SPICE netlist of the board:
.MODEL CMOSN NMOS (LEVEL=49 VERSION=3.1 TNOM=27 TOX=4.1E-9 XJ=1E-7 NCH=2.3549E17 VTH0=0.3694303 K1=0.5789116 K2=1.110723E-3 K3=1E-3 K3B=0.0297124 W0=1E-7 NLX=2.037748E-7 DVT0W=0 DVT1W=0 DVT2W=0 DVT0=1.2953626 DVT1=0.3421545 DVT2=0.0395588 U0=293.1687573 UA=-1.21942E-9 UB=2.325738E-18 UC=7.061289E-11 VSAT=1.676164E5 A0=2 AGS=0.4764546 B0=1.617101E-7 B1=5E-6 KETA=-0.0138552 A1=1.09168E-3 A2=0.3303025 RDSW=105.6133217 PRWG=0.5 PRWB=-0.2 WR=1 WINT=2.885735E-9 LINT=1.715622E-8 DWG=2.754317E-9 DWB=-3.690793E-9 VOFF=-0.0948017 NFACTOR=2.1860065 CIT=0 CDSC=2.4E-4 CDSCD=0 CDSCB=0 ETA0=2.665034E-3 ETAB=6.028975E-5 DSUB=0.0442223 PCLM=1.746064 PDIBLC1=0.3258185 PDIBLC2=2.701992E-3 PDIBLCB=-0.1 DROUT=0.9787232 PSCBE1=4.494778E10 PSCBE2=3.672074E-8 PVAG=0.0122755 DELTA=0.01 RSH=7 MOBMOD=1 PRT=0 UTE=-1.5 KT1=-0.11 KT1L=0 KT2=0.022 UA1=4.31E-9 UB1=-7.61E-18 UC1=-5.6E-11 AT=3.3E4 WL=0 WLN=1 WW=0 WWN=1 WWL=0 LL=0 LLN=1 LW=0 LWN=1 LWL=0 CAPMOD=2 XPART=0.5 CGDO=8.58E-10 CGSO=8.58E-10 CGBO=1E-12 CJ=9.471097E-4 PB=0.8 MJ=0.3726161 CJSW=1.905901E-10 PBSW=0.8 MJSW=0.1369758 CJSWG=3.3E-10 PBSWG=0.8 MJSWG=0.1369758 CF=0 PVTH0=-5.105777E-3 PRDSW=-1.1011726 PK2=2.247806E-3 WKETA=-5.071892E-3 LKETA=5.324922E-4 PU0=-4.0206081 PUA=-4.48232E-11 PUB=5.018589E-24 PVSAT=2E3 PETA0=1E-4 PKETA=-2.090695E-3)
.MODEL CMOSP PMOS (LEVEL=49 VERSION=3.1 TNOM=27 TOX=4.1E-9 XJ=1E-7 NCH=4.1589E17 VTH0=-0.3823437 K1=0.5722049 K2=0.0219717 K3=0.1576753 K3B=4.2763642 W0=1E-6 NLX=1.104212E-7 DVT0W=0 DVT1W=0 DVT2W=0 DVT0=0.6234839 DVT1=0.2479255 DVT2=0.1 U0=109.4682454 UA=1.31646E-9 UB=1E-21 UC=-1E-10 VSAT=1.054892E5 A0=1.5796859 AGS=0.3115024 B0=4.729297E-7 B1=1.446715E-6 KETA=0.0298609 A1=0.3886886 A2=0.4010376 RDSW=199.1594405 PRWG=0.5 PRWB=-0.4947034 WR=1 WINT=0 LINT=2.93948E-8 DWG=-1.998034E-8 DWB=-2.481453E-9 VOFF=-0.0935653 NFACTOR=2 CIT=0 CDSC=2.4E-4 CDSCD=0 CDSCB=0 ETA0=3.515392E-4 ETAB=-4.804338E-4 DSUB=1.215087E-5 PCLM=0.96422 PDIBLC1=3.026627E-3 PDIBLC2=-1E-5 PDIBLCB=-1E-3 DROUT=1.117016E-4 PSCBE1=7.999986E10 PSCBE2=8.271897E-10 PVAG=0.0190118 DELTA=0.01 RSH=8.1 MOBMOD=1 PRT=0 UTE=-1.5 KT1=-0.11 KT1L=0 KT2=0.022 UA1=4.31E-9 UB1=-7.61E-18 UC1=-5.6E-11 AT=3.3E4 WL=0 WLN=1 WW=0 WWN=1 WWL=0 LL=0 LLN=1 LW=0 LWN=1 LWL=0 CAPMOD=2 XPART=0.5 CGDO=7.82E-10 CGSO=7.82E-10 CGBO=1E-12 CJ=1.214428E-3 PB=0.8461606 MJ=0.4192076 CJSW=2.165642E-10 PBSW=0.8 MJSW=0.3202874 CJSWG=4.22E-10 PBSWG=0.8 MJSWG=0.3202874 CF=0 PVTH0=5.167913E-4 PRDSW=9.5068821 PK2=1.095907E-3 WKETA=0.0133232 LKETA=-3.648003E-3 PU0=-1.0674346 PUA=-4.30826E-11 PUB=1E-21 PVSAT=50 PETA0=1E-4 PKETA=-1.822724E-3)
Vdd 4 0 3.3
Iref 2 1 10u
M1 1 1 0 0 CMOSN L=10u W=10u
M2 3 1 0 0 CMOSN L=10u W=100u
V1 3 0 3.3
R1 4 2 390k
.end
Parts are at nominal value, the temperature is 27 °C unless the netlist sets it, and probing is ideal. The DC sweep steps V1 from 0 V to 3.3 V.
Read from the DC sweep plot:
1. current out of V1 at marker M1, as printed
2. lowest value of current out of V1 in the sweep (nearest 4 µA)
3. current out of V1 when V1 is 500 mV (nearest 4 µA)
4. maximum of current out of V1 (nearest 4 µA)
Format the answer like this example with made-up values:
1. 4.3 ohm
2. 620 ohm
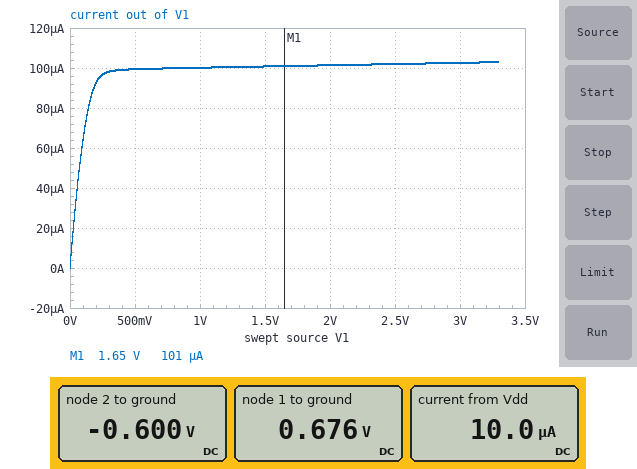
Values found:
1. 101 µA
2. 0 A
3. 100 µA
4. 104 µA
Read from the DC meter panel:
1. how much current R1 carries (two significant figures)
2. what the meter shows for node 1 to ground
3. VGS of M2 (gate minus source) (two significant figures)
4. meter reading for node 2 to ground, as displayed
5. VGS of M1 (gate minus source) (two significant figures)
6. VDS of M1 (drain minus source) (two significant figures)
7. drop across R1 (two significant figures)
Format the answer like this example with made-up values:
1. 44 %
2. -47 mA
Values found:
1. 10 µA
2. 0.676 V
3. 680 mV
4. -0.600 V
5. 680 mV
6. 680 mV
7. 3.9 V
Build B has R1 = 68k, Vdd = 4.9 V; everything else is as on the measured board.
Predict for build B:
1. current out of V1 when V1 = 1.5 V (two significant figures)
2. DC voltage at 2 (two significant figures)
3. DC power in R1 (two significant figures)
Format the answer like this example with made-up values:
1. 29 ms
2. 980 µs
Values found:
1. 100 µA
2. 4.2 V
3. 6.8 µW
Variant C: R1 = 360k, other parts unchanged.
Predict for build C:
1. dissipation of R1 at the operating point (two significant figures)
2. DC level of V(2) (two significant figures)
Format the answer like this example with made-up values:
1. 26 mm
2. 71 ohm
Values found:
1. 36 µW
2. -300 mV
